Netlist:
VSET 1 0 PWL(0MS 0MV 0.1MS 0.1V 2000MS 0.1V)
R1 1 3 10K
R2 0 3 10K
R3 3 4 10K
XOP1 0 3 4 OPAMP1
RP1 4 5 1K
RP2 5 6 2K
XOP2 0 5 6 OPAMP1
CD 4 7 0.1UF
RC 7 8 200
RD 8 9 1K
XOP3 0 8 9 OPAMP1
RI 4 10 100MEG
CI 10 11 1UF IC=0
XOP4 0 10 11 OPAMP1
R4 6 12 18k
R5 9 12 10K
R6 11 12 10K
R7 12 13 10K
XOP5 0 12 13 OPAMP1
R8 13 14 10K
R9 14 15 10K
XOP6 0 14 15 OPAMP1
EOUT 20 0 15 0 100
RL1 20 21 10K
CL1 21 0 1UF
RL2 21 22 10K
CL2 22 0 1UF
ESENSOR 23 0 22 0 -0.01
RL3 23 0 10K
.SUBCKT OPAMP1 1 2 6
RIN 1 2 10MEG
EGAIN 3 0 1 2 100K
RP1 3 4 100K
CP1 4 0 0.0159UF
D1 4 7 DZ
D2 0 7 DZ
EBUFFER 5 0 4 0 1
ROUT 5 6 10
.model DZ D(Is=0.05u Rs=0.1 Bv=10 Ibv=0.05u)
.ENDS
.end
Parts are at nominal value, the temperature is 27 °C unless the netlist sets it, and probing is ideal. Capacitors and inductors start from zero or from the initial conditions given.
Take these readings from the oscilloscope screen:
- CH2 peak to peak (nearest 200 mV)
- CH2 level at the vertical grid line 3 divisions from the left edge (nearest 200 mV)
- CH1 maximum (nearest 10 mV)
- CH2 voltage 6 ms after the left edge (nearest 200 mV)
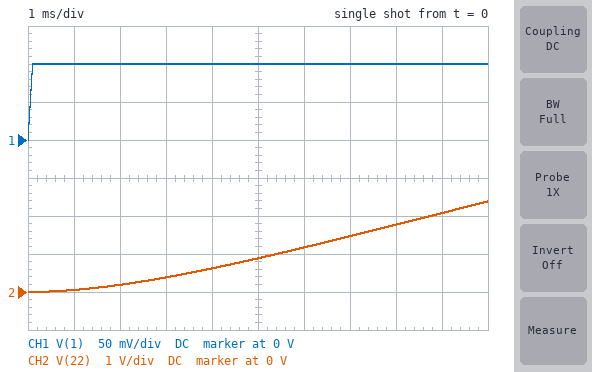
2.4 V
400 mV
100 mV
1.2 V
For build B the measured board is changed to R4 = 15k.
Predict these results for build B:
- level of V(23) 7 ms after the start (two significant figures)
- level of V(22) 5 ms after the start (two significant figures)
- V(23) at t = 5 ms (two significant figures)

-18 mV
1.1 V
-11 mV
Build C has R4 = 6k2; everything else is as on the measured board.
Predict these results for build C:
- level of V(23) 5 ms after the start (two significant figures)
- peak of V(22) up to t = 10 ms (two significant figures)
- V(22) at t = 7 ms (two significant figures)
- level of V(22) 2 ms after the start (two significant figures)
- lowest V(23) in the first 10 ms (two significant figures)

-25 mV
6.9 V
4.2 V
520 mV
-69 mV
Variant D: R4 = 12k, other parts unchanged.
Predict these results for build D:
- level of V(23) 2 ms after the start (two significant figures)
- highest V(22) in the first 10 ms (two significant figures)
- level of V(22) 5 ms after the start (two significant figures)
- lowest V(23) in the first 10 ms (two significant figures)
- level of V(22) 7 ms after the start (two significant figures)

-2.8 mV
3.6 V
1.3 V
-36 mV
2.2 V
